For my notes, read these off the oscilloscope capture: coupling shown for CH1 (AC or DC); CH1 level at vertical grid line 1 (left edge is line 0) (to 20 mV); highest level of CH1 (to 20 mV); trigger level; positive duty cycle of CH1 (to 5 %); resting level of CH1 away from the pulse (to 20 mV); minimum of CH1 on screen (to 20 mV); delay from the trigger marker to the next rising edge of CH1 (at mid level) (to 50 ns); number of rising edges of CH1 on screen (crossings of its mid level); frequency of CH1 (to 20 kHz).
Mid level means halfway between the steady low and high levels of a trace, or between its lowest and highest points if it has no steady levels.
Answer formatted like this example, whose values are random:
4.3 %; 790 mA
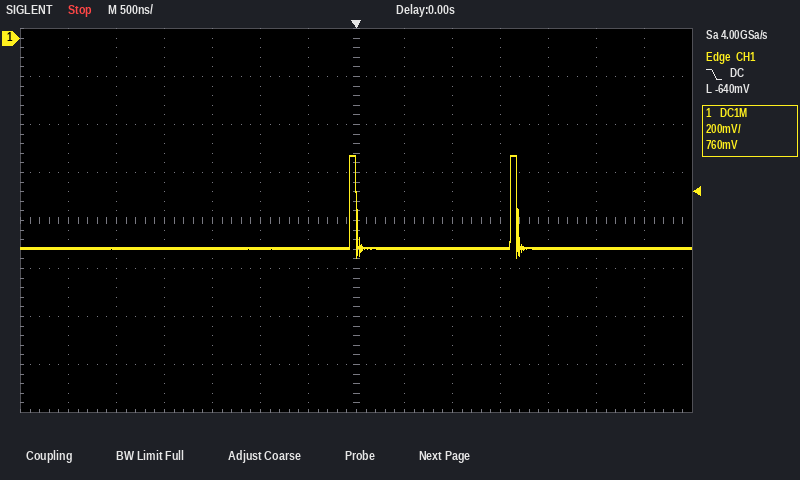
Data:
DC; -880 mV; -480 mV; -640 mV; 5 %; -880 mV; -920 mV; 1.60 µs; 2; 600 kHz
